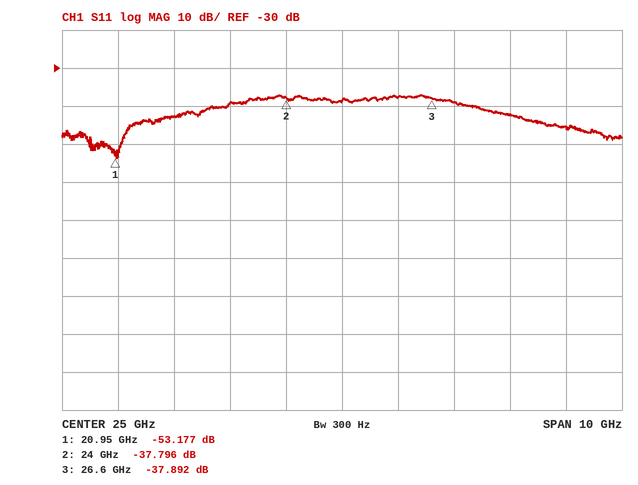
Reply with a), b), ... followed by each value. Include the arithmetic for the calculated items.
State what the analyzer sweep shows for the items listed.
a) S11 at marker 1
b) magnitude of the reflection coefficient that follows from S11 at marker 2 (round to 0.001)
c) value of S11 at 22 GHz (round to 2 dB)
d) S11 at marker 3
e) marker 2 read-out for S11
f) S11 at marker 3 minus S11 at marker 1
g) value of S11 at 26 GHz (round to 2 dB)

a) -53.177 dB
b) 10^(-37.796/20) ≈ 0.013
c) -42 dB
d) -37.892 dB
e) -37.796 dB
f) -37.892 − (-53.177) = 15.285 dB
g) -38 dB
